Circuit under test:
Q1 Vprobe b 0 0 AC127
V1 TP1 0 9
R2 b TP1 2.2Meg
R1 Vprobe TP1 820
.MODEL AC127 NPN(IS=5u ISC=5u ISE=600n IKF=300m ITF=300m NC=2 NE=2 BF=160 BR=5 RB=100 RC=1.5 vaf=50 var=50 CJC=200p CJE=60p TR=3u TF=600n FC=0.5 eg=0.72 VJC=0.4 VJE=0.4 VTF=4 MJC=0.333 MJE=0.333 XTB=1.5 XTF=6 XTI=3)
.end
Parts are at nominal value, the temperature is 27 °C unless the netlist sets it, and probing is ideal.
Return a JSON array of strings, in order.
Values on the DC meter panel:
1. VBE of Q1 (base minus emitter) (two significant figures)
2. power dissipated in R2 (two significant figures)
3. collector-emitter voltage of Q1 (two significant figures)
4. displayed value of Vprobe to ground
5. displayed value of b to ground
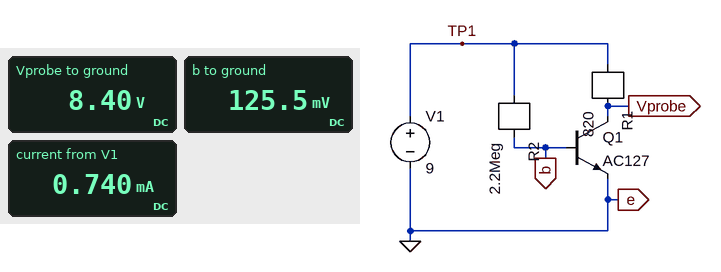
["130 mV", "36 µW", "8.4 V", "8.40 V", "125.5 mV"]
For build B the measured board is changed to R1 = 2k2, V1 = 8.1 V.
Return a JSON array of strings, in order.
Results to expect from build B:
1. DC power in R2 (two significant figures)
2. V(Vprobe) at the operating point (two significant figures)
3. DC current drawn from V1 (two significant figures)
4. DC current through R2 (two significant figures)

["29 µW", "6.6 V", "680 µA", "3.6 µA"]
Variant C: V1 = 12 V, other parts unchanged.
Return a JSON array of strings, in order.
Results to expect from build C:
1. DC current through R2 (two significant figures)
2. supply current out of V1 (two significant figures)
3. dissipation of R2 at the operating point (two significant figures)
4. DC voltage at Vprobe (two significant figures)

["5.4 µA", "920 µA", "64 µW", "11 V"]
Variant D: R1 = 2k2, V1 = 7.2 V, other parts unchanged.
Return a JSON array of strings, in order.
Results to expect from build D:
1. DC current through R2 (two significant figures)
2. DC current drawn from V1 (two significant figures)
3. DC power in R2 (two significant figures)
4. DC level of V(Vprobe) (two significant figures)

["3.2 µA", "630 µA", "23 µW", "5.8 V"]
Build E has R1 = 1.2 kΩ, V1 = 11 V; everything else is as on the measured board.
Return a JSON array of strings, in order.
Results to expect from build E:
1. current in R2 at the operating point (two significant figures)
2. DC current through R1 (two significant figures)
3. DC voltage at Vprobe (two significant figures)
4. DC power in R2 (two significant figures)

["4.9 µA", "850 µA", "10 V", "54 µW"]
